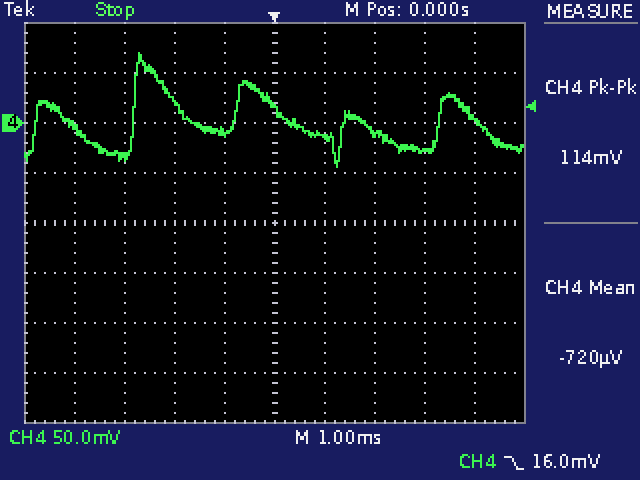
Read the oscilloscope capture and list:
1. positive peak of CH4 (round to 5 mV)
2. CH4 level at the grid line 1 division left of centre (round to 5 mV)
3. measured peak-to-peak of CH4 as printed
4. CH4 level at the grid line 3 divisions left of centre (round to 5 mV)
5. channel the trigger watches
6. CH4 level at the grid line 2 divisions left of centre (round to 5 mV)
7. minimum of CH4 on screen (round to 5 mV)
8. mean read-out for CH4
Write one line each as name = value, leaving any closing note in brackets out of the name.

positive peak of CH4 = 70 mV
CH4 level at the grid line 1 division left of centre = -10 mV
measured peak-to-peak of CH4 as printed = 114 mV
CH4 level at the grid line 3 divisions left of centre = -35 mV
channel the trigger watches = CH4
CH4 level at the grid line 2 divisions left of centre = 20 mV
minimum of CH4 on screen = -45 mV
mean read-out for CH4 = -720 µV
